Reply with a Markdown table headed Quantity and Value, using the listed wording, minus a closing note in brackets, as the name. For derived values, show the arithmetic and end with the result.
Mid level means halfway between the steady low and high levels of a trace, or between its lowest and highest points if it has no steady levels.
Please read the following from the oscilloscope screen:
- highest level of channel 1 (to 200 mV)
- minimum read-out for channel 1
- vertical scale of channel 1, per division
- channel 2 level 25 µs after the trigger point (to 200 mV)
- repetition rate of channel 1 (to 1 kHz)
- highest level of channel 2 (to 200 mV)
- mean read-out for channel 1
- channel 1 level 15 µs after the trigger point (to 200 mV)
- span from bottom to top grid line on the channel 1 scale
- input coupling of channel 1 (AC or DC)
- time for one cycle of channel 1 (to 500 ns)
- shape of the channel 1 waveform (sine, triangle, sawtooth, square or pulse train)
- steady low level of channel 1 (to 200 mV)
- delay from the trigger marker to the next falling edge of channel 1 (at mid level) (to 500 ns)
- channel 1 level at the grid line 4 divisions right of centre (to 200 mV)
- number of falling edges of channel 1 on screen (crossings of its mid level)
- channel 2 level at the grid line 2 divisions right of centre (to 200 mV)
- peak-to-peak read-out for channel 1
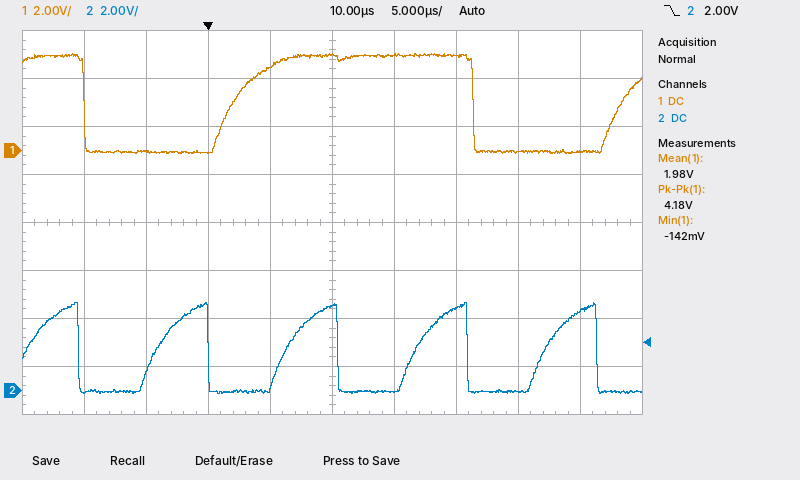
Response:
| Quantity | Value |
|---|---|
| highest level of channel 1 | 4.0 V |
| minimum read-out for channel 1 | -142 mV |
| vertical scale of channel 1, per division | 2 V |
| channel 2 level 25 µs after the trigger point | 0.0 V |
| repetition rate of channel 1 | 1 / 31.5 µs ≈ 32 kHz |
| highest level of channel 2 | 3.6 V |
| mean read-out for channel 1 | 1.98 V |
| channel 1 level 15 µs after the trigger point | 4.0 V |
| span from bottom to top grid line on the channel 1 scale | 16 V |
| input coupling of channel 1 | DC |
| time for one cycle of channel 1 | 31.5 µs |
| shape of the channel 1 waveform | pulse train |
| steady low level of channel 1 | 0.0 V |
| delay from the trigger marker to the next falling edge of channel 1 (at mid level) | 21.5 µs |
| channel 1 level at the grid line 4 divisions right of centre | 0.0 V |
| number of falling edges of channel 1 on screen | 2 |
| channel 2 level at the grid line 2 divisions right of centre | 3.4 V |
| peak-to-peak read-out for channel 1 | 4.18 V |
